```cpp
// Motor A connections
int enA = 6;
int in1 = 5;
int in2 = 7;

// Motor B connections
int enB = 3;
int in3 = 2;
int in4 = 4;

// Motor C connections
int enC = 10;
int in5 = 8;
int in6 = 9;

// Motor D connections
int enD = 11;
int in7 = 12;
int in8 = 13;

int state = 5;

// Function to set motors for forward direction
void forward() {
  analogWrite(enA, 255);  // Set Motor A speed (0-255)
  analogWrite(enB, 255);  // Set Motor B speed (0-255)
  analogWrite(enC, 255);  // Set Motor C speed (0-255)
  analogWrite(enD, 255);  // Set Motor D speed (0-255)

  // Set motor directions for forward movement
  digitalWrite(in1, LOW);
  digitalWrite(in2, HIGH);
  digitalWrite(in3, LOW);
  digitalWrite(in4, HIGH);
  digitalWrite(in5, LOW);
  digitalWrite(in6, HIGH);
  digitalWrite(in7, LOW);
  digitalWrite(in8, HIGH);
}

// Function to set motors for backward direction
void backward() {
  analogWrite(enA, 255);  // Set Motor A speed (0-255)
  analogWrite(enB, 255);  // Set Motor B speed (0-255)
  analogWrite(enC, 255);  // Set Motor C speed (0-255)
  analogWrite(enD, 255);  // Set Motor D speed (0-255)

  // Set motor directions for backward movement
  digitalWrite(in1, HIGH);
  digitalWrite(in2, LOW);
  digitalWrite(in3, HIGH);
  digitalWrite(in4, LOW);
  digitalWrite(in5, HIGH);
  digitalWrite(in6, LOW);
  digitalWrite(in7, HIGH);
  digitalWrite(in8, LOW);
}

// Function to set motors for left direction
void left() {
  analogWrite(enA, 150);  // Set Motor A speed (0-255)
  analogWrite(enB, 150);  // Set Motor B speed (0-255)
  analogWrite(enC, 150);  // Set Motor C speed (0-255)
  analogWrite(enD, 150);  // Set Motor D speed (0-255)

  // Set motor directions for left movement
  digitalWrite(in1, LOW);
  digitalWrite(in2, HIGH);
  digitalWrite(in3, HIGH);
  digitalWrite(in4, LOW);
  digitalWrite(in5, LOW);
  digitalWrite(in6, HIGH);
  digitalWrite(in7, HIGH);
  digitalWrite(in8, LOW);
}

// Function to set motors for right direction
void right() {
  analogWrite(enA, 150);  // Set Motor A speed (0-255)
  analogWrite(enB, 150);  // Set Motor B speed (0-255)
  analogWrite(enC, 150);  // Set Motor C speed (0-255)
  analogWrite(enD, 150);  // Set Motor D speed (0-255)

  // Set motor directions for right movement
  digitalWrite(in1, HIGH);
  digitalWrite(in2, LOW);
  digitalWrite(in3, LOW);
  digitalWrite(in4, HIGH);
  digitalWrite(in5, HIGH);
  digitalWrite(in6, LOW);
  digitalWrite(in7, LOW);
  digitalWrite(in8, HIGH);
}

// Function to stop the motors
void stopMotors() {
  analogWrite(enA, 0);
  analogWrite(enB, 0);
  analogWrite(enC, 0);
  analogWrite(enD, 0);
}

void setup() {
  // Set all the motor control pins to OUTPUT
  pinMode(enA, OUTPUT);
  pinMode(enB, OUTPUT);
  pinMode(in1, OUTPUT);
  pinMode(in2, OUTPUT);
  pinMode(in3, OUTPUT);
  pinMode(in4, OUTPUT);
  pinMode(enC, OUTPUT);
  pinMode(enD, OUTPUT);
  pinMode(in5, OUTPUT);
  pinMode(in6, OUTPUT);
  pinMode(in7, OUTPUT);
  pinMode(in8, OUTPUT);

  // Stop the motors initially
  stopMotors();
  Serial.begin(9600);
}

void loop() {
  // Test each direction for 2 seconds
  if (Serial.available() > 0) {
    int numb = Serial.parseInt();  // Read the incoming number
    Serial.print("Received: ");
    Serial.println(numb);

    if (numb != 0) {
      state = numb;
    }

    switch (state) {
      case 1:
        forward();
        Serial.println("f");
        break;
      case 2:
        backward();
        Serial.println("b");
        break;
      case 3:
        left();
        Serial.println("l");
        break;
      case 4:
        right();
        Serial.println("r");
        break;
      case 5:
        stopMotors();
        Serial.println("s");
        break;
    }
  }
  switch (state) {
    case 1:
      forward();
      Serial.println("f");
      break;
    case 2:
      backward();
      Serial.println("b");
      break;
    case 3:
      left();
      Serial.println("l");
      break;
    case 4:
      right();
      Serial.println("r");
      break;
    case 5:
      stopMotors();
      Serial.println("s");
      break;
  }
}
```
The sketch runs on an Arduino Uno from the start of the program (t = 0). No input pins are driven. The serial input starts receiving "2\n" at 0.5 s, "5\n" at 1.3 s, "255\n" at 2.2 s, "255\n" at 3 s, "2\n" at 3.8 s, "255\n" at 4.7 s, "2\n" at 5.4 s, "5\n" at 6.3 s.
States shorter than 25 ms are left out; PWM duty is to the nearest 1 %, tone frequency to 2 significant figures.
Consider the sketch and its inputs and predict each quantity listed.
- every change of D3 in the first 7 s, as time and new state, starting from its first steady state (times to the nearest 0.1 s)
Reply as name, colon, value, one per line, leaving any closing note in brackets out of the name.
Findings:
every change of D3 in the first 7 s, as time and new state, starting from its first steady state: 0 s low; 0.5 s high; 1.3 s low; 3.8 s high; 6.3 s low
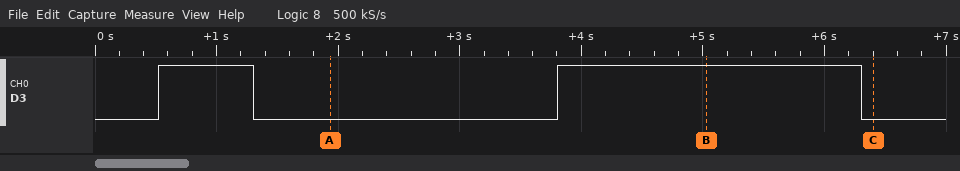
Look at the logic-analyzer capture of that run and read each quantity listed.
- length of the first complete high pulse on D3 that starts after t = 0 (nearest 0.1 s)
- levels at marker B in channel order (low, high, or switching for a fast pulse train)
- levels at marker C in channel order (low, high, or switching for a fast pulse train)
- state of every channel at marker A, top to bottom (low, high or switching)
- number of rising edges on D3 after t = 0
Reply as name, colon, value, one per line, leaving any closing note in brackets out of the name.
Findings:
length of the first complete high pulse on D3 that starts after t = 0: 0.8 s
levels at marker B in channel order: D3 high
levels at marker C in channel order: D3 low
state of every channel at marker A, top to bottom: D3 low
number of rising edges on D3 after t = 0: 2
